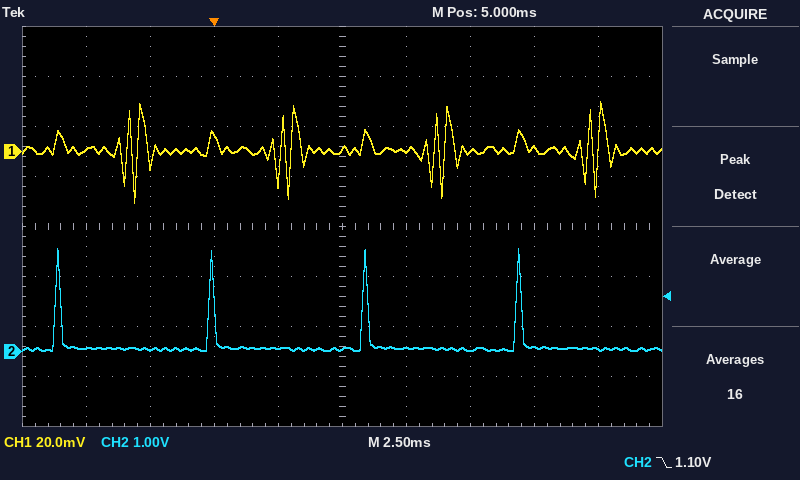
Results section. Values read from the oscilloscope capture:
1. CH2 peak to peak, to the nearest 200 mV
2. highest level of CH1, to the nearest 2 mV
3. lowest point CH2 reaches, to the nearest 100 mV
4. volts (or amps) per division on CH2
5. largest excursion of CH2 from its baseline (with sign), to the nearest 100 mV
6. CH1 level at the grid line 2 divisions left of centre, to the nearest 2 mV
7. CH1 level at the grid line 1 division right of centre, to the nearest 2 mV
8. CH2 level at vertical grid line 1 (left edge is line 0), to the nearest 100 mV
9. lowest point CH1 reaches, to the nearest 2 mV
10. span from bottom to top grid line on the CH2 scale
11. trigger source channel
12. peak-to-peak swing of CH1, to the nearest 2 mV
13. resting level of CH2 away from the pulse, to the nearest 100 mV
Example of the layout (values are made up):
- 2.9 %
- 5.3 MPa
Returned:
- 2.0 V
- 20 mV
- 0.0 V
- 1 V
- +2.0 V
- 6 mV
- 0 mV
- 100 mV
- -20 mV
- 8 V
- CH2
- 40 mV
- 100 mV
